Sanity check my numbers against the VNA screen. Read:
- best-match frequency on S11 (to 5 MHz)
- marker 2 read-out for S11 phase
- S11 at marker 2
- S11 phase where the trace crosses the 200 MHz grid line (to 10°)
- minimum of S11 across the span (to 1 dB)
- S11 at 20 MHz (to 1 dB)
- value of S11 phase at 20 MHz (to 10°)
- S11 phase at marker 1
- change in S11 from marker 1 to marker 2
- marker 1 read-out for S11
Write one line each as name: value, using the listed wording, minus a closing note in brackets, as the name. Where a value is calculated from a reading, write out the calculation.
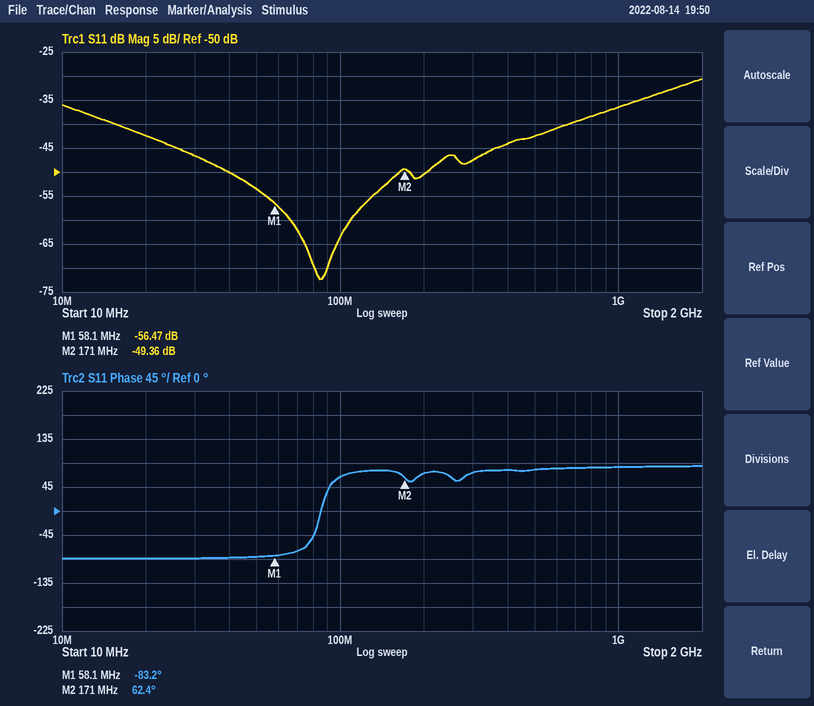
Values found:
best-match frequency on S11: 85 MHz
marker 2 read-out for S11 phase: 62.4°
S11 at marker 2: -49.36 dB
S11 phase where the trace crosses the 200 MHz grid line: 70°
minimum of S11 across the span: -72 dB
S11 at 20 MHz: -42 dB
value of S11 phase at 20 MHz: -90°
S11 phase at marker 1: -83.2°
change in S11 from marker 1 to marker 2: -49.36 − (-56.47) = 7.11 dB
marker 1 read-out for S11: -56.47 dB
